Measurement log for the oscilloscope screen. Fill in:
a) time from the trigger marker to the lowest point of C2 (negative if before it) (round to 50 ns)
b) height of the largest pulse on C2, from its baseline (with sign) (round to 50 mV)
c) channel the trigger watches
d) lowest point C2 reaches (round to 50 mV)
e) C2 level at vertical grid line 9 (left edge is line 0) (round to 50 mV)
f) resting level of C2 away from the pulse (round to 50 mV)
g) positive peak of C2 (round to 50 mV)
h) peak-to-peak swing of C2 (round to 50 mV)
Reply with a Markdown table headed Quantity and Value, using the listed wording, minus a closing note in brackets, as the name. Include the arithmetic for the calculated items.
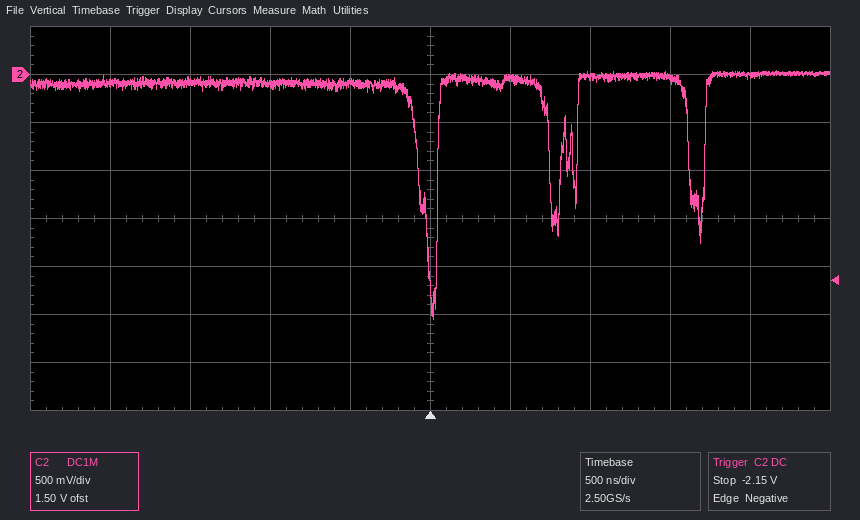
| Quantity | Value |
|---|---|
| time from the trigger marker to the lowest point of C2 (negative if before it) | 0 ns |
| height of the largest pulse on C2, from its baseline (with sign) | -2.55 V − (-100 mV) = -2.45 V |
| channel the trigger watches | C2 |
| lowest point C2 reaches | -2.55 V |
| C2 level at vertical grid line 9 (left edge is line 0) | 0 mV |
| resting level of C2 away from the pulse | -100 mV |
| positive peak of C2 | 50 mV |
| peak-to-peak swing of C2 | 50 mV − (-2.55 V) = 2.60 V |
